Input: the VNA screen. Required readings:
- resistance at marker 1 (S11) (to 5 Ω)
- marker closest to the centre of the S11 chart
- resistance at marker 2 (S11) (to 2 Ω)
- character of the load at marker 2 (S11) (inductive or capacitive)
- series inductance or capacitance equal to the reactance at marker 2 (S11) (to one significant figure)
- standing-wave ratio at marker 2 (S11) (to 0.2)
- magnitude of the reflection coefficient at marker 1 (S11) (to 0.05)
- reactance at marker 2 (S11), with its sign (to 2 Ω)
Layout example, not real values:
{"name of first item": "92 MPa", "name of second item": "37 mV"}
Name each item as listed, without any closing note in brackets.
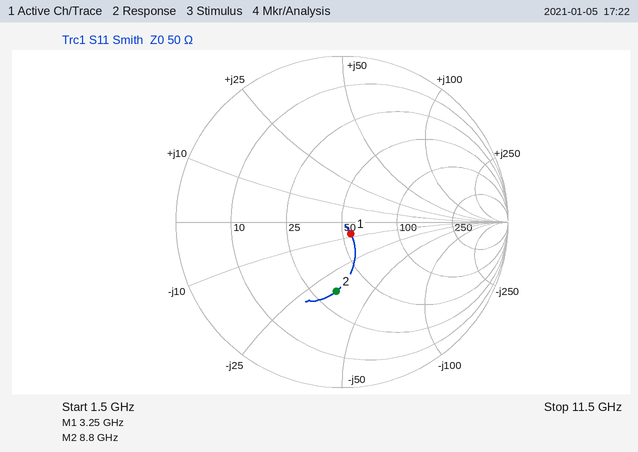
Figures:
{"resistance at marker 1 (S11)": "55 Ω", "marker closest to the centre of the S11 chart": "marker 1", "resistance at marker 2 (S11)": "34 Ω", "character of the load at marker 2 (S11)": "capacitive", "series inductance or capacitance equal to the reactance at marker 2 (S11)": "500 fF", "standing-wave ratio at marker 2 (S11)": "2.4", "magnitude of the reflection coefficient at marker 1 (S11)": "0.10", "reactance at marker 2 (S11), with its sign": "-34 Ω"}
